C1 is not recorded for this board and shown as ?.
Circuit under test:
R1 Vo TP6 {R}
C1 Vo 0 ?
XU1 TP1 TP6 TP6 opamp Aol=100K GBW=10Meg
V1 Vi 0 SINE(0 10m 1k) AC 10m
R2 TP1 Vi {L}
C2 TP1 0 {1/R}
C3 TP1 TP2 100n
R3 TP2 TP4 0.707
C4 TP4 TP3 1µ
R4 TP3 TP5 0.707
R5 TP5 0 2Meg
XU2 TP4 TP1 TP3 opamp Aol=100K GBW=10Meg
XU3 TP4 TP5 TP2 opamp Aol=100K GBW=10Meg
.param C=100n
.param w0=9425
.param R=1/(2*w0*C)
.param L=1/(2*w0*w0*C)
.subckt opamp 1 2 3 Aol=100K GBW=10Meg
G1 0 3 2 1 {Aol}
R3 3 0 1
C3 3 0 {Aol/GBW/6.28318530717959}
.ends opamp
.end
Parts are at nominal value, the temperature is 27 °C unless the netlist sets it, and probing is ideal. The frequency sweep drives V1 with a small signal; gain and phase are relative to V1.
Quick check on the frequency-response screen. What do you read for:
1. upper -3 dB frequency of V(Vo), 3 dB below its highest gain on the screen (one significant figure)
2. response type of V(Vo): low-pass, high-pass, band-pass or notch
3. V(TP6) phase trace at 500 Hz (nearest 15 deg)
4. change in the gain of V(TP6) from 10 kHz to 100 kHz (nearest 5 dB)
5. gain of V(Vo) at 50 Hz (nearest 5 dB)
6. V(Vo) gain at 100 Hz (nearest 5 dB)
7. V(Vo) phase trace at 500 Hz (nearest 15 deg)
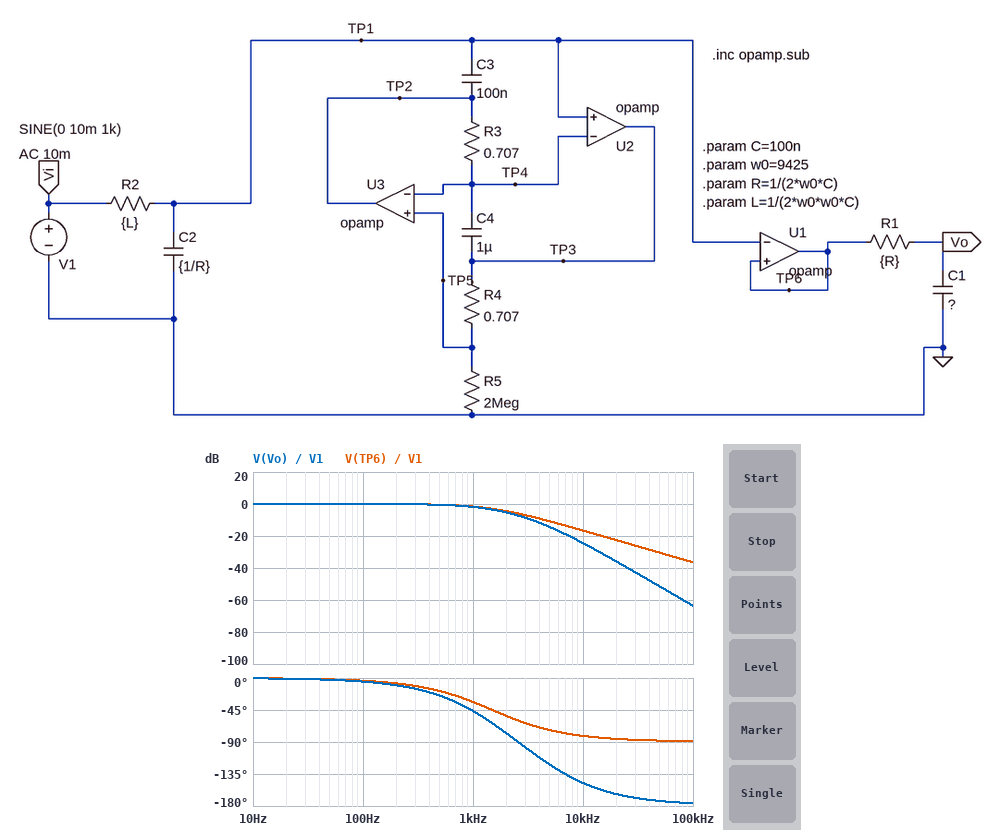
1 kHz
low-pass
-15 deg
-20 dB
0 dB
0 dB
-30 deg
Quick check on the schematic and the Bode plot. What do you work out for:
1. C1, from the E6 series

68 nF
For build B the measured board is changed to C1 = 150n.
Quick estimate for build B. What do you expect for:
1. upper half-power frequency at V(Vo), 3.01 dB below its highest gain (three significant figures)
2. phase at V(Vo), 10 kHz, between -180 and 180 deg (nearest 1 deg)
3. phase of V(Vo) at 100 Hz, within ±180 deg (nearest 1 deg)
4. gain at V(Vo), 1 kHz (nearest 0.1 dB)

1.10 kHz
-160 deg
-7 deg
-2.6 dB
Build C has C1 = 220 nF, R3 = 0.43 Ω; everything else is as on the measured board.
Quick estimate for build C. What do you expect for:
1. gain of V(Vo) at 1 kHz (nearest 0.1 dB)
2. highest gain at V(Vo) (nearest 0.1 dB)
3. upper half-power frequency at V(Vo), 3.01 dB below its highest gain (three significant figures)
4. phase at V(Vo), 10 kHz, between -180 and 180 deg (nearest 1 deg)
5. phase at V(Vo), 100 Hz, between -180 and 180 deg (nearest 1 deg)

-3.5 dB
0 dB
919 Hz
-164 deg
-8 deg
